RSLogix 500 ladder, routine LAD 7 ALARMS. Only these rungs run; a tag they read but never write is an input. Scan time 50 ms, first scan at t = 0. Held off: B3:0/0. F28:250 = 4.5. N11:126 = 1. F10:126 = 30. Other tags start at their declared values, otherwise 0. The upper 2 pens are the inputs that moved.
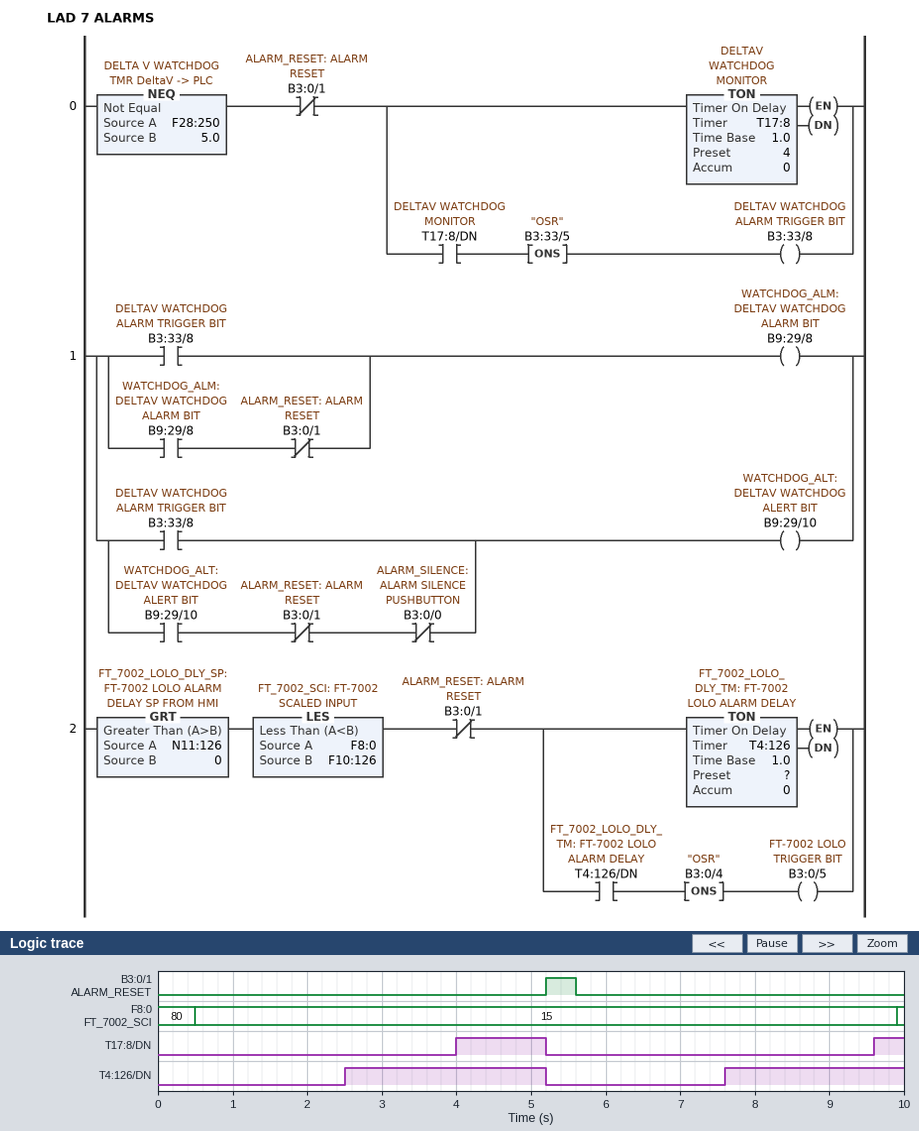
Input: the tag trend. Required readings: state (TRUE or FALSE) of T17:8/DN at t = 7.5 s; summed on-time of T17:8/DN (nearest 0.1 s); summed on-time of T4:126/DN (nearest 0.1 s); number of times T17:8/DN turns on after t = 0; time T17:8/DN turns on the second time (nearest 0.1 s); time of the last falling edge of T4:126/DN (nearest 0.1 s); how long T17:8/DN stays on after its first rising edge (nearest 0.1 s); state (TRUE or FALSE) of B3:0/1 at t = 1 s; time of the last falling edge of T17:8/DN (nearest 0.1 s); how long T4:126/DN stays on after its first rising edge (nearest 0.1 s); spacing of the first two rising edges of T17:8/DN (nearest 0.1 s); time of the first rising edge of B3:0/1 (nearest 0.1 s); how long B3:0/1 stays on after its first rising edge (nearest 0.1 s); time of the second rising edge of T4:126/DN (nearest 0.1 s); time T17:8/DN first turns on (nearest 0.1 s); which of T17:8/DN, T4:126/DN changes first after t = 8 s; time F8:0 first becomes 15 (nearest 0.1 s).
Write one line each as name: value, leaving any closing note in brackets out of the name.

state (TRUE or FALSE) of T17:8/DN at t = 7.5 s: FALSE
summed on-time of T17:8/DN: 1.6 s
summed on-time of T4:126/DN: 5.1 s
number of times T17:8/DN turns on after t = 0: 2
time T17:8/DN turns on the second time: 9.6 s
time of the last falling edge of T4:126/DN: 5.2 s
how long T17:8/DN stays on after its first rising edge: 1.2 s
state (TRUE or FALSE) of B3:0/1 at t = 1 s: FALSE
time of the last falling edge of T17:8/DN: 5.2 s
how long T4:126/DN stays on after its first rising edge: 2.7 s
spacing of the first two rising edges of T17:8/DN: 5.6 s
time of the first rising edge of B3:0/1: 5.2 s
how long B3:0/1 stays on after its first rising edge: 0.4 s
time of the second rising edge of T4:126/DN: 7.6 s
time T17:8/DN first turns on: 4.0 s
which of T17:8/DN, T4:126/DN changes first after t = 8 s: T17:8/DN
time F8:0 first becomes 15: 0.5 s
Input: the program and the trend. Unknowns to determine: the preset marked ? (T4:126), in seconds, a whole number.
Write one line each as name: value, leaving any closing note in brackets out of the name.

the preset marked ? (T4:126), in seconds, a whole number: 2 s
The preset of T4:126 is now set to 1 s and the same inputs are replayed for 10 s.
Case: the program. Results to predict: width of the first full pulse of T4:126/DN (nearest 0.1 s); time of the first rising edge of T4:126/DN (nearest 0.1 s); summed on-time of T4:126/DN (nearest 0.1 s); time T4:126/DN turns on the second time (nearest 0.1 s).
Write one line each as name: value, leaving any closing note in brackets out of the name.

width of the first full pulse of T4:126/DN: 3.7 s
time of the first rising edge of T4:126/DN: 1.5 s
summed on-time of T4:126/DN: 7.1 s
time T4:126/DN turns on the second time: 6.6 s
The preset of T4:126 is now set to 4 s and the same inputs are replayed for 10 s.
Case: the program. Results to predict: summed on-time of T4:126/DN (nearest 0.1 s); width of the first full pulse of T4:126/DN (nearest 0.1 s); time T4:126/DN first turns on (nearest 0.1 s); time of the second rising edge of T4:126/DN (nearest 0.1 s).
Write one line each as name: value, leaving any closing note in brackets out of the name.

summed on-time of T4:126/DN: 1.1 s
width of the first full pulse of T4:126/DN: 0.7 s
time T4:126/DN first turns on: 4.5 s
time of the second rising edge of T4:126/DN: 9.6 s
